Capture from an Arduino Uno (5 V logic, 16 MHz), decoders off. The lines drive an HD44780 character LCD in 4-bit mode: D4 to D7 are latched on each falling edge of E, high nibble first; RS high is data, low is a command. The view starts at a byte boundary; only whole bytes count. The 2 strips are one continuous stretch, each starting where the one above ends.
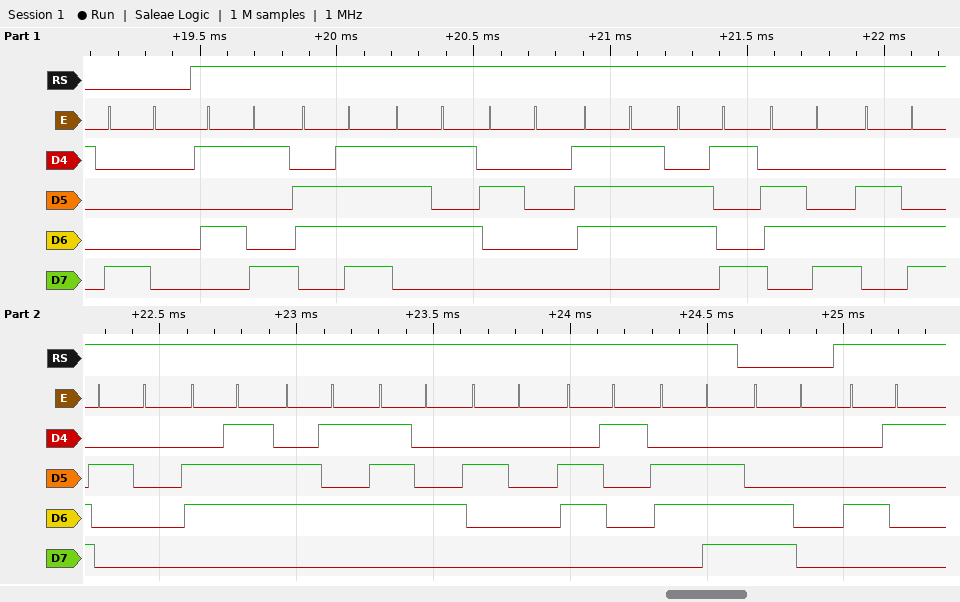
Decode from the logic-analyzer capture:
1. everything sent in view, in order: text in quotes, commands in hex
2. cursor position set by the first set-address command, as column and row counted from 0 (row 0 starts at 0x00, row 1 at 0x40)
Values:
0x80 "You will get an" 0xC0 "A"
column 0, row 0
